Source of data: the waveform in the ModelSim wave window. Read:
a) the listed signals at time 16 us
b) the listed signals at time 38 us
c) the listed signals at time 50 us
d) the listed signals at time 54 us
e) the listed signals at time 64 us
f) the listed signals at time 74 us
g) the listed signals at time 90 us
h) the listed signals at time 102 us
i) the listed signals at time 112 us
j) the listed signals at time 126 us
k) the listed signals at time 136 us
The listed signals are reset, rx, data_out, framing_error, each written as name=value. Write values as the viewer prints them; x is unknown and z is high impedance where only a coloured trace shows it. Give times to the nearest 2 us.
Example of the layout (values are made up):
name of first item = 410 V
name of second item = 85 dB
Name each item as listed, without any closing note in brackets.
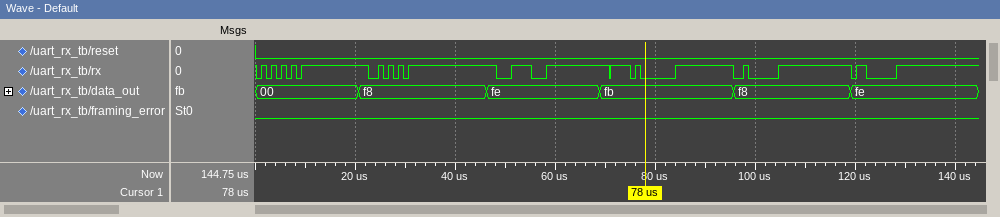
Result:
the listed signals at time 16 us = reset=0, rx=1, data_out=00, framing_error=0
the listed signals at time 38 us = reset=0, rx=1, data_out=f8, framing_error=0
the listed signals at time 50 us = reset=0, rx=0, data_out=fe, framing_error=0
the listed signals at time 54 us = reset=0, rx=1, data_out=fe, framing_error=0
the listed signals at time 64 us = reset=0, rx=1, data_out=fe, framing_error=0
the listed signals at time 74 us = reset=0, rx=1, data_out=fb, framing_error=0
the listed signals at time 90 us = reset=0, rx=1, data_out=fb, framing_error=0
the listed signals at time 102 us = reset=0, rx=0, data_out=f8, framing_error=0
the listed signals at time 112 us = reset=0, rx=1, data_out=f8, framing_error=0
the listed signals at time 126 us = reset=0, rx=0, data_out=fe, framing_error=0
the listed signals at time 136 us = reset=0, rx=1, data_out=fe, framing_error=0
